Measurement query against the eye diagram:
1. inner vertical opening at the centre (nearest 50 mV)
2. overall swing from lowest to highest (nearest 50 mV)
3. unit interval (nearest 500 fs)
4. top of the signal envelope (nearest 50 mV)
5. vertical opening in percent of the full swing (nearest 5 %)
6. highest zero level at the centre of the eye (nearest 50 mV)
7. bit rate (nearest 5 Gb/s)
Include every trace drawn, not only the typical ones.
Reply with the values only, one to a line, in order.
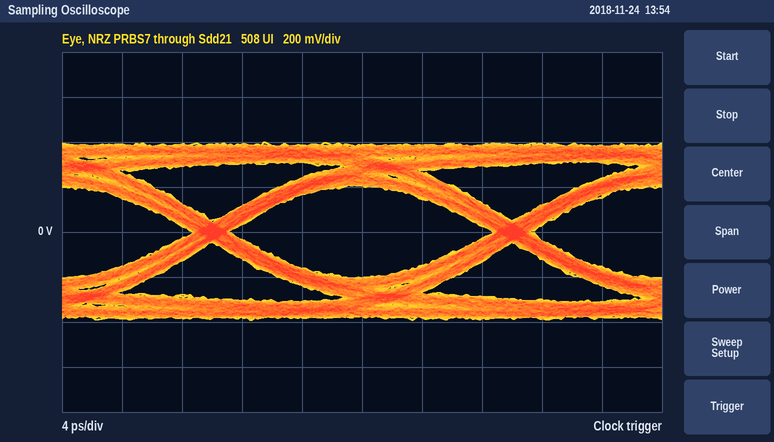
400 mV
800 mV
20.0 ps
400 mV
50 %
-200 mV
50 Gb/s
